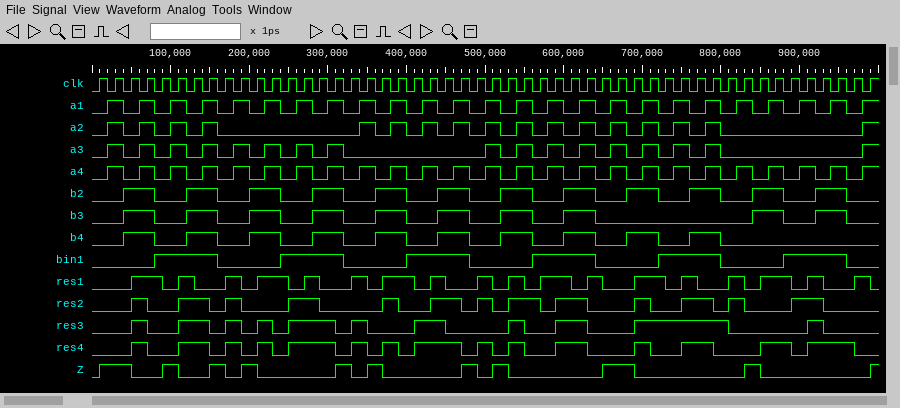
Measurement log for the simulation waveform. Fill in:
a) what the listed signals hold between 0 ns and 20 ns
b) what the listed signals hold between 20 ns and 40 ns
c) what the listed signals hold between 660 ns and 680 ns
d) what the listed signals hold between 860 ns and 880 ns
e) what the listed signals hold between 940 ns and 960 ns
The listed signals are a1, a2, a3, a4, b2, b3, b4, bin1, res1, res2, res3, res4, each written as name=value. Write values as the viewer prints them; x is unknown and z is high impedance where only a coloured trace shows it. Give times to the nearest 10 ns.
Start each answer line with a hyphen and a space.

- a1=0, a2=0, a3=0, a4=0, b2=0, b3=0, b4=0, bin1=0, res1=0, res2=0, res3=0, res4=0
- a1=1, a2=1, a3=1, a4=1, b2=0, b3=0, b4=0, bin1=0, res1=0, res2=0, res3=0, res4=0
- a1=1, a2=1, a3=1, a4=1, b2=0, b3=0, b4=0, bin1=0, res1=0, res2=0, res3=0, res4=0
- a1=1, a2=0, a3=0, a4=1, b2=1, b3=1, b4=0, bin1=0, res1=1, res2=0, res3=0, res4=1
- a1=1, a2=0, a3=0, a4=1, b2=1, b3=1, b4=0, bin1=1, res1=0, res2=0, res3=0, res4=1
